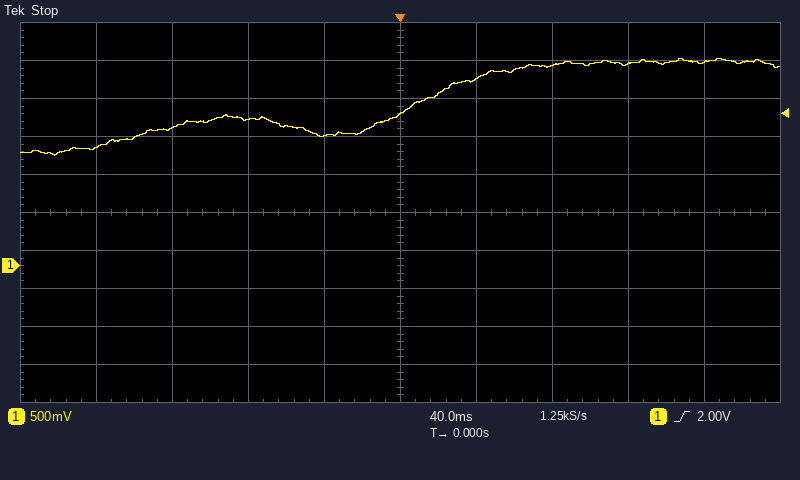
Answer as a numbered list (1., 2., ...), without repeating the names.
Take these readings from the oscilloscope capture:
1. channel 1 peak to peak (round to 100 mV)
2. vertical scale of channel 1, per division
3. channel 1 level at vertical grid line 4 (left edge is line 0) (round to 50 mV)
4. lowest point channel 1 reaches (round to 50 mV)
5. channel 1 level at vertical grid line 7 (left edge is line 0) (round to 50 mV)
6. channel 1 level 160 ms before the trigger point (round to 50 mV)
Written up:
1. 1.30 V
2. 500 mV
3. 1.70 V
4. 1.45 V
5. 2.65 V
6. 1.55 V
